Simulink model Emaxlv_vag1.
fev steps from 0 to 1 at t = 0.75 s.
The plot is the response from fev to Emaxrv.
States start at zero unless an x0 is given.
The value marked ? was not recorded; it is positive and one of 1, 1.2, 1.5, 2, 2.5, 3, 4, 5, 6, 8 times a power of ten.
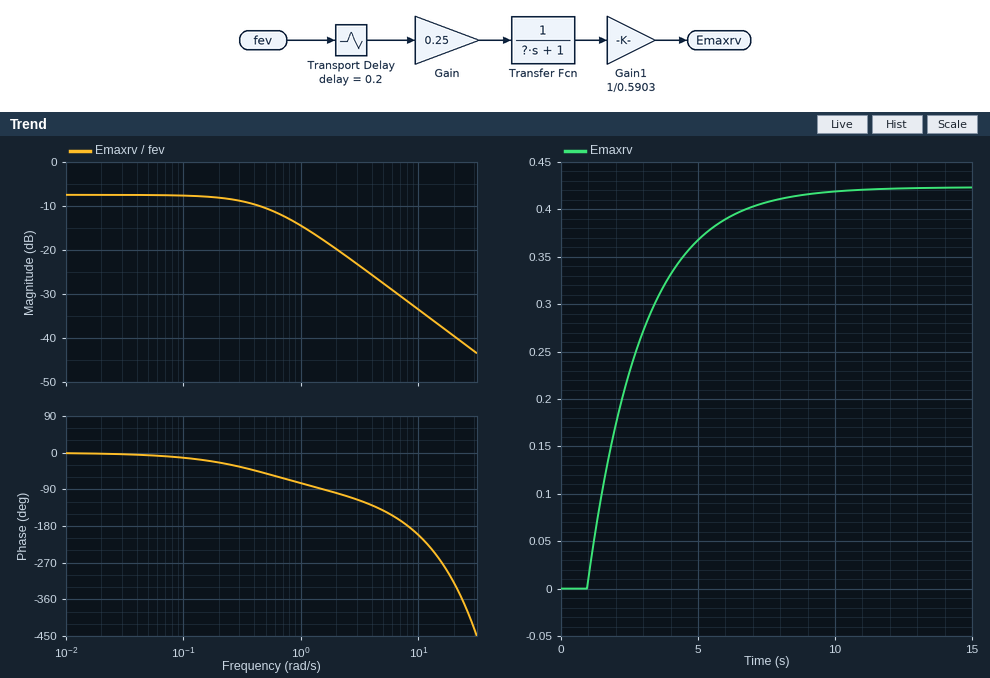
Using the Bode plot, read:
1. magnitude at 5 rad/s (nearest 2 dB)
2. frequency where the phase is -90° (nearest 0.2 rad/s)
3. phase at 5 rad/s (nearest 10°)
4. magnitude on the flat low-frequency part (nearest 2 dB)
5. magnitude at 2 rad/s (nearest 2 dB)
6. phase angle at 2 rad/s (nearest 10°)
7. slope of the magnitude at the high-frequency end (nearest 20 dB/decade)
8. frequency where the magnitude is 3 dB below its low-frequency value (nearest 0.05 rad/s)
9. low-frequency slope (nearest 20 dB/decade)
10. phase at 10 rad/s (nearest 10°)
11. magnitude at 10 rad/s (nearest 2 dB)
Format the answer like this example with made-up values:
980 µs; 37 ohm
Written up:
-28 dB; 1.6 rad/s; -140°; -8 dB; -20 dB; -100°; -20 dB/decade; 0.50 rad/s; 0 dB/decade; -200°; -34 dB
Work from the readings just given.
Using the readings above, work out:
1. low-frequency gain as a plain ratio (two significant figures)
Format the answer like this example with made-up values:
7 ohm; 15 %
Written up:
0.40
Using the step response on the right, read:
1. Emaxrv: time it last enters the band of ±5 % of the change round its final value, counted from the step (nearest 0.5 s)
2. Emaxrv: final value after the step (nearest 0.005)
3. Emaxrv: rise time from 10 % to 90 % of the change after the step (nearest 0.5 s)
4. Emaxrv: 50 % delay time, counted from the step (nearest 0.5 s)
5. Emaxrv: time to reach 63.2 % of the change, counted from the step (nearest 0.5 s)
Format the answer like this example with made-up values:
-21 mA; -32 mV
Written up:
6.0 s; 0.425; 4.5 s; 1.5 s; 2.0 s
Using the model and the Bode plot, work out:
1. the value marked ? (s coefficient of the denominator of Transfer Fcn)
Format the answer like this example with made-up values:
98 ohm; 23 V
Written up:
2
